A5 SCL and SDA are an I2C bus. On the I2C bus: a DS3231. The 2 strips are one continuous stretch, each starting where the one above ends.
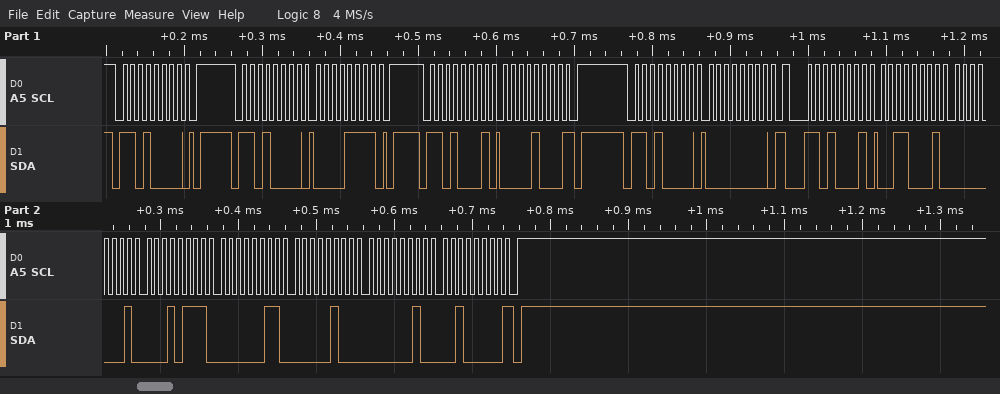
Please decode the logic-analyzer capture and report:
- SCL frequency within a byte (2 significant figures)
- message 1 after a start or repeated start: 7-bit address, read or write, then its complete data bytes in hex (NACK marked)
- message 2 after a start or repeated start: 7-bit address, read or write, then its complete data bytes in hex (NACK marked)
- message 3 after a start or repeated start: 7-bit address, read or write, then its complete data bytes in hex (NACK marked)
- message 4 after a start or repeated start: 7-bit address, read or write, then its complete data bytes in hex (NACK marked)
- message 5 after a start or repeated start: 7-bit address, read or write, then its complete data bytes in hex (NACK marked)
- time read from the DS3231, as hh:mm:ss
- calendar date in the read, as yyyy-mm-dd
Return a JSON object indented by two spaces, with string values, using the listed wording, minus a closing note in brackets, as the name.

{
  "SCL frequency within a byte": "100 kHz",
  "message 1 after a start or repeated start: 7-bit address, read or write, then its complete data bytes in hex": "0x68 write",
  "message 2 after a start or repeated start: 7-bit address, read or write, then its complete data bytes in hex": "0x68 write: 0F",
  "message 3 after a start or repeated start: 7-bit address, read or write, then its complete data bytes in hex": "0x68 read: 08 NACK",
  "message 4 after a start or repeated start: 7-bit address, read or write, then its complete data bytes in hex": "0x68 write: 00",
  "message 5 after a start or repeated start: 7-bit address, read or write, then its complete data bytes in hex": "0x68 read: 31 01 17 03 04 02 20 NACK",
  "time read from the DS3231, as hh:mm:ss": "17:01:31",
  "calendar date in the read, as yyyy-mm-dd": "2020-02-04"
}
